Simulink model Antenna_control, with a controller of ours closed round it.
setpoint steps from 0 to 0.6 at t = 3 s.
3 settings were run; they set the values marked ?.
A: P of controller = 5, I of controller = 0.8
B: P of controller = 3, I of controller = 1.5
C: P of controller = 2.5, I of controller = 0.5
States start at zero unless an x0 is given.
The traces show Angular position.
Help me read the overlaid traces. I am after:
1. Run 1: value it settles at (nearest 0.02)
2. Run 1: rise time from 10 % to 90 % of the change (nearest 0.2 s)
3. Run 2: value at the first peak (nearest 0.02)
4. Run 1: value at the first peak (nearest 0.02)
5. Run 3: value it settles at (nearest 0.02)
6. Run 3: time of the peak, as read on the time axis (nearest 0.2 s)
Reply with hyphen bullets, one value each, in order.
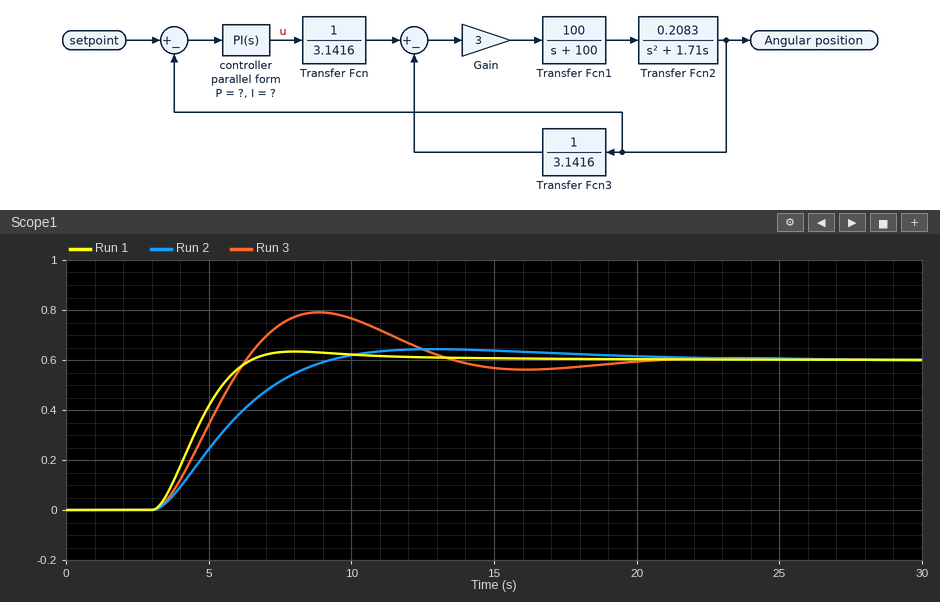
- 0.60
- 2.2 s
- 0.64
- 0.64
- 0.60
- 8.8 s
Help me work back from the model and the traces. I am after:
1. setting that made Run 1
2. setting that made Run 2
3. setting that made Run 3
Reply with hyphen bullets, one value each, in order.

- A
- C
- B
